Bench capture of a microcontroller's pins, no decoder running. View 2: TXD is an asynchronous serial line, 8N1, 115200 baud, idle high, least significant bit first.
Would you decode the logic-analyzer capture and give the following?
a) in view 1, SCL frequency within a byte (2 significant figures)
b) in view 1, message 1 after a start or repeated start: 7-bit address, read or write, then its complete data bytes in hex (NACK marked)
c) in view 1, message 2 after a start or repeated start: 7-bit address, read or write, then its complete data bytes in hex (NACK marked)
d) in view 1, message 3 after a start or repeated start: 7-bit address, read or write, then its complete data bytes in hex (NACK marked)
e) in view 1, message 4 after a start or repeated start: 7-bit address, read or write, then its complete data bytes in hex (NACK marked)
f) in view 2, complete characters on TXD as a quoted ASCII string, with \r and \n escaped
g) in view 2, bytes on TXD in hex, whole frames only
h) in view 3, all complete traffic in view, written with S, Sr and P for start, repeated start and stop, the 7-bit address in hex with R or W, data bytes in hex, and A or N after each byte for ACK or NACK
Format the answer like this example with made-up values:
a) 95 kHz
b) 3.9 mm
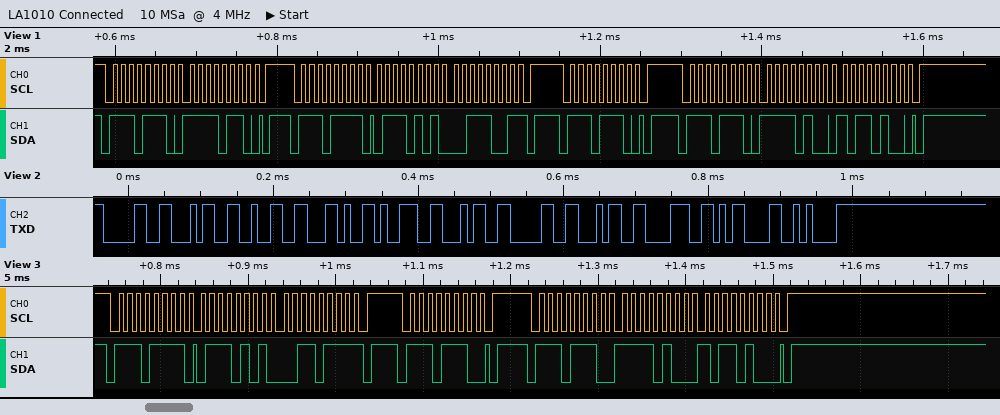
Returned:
a) 100 kHz
b) 0x77 write: F6
c) 0x77 read: 75 39 NACK
d) 0x77 write
e) 0x77 write: F4 B4
f) "042,94048\r\n"
g) 30 34 32 2C 39 34 30 34 38 0D 0A
h) S 77R A 75 A 37 N P S 77W A P S 77W A F4 A B4 A P
